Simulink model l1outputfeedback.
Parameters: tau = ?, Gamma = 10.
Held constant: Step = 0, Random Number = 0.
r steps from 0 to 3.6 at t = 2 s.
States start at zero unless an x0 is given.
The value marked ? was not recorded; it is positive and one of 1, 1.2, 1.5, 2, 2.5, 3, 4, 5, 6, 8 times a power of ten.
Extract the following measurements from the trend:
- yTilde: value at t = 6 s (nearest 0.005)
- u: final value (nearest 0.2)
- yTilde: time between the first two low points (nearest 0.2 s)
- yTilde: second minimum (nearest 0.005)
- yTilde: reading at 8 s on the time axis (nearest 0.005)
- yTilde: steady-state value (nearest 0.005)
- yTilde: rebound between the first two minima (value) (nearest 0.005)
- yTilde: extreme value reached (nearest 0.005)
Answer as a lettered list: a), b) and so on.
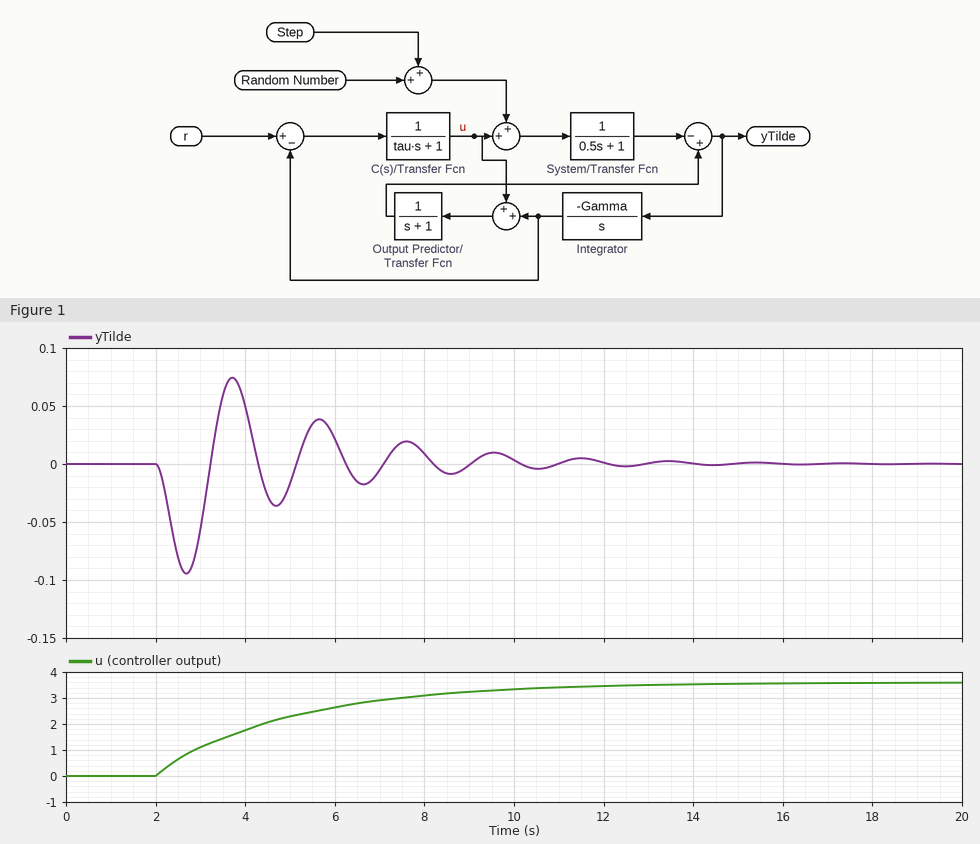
a) 0.020
b) 3.6
c) 2.0 s
d) -0.035
e) 0.010
f) 0.000
g) 0.075
h) -0.095
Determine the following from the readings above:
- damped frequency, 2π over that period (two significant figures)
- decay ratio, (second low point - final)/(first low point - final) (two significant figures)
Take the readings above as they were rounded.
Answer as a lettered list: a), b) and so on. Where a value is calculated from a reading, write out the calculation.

a) 2π / 2 = 3.1 rad/s
b) (-0.035 - 0) / (-0.095 - 0) = 0.37
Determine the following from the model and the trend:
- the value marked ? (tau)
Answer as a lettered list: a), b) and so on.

a) 2.5
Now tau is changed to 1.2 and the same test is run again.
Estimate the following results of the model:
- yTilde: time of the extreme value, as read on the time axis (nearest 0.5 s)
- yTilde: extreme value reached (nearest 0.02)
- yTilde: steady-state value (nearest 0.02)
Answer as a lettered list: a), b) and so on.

a) 2.5 s
b) -0.16
c) 0.00
